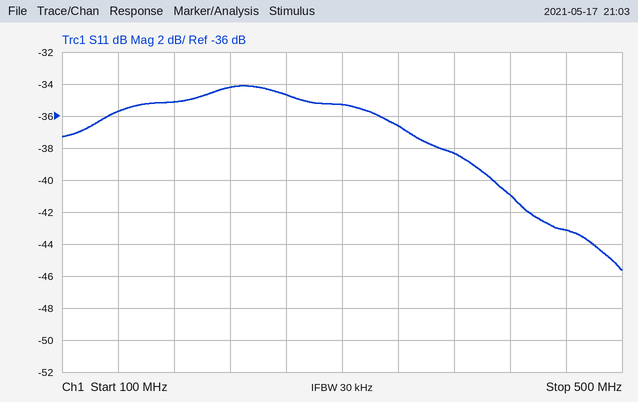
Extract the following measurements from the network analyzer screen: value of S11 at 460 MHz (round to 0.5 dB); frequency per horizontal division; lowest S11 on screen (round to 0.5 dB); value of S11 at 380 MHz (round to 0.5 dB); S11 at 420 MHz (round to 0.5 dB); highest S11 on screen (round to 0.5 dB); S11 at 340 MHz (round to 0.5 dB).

-43.0 dB
40 MHz
-45.5 dB
-38.5 dB
-41.0 dB
-34.0 dB
-36.5 dB
